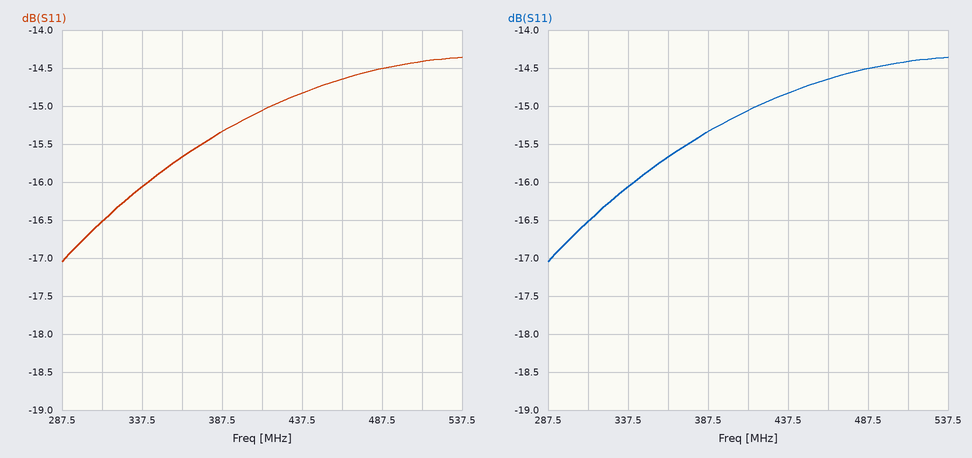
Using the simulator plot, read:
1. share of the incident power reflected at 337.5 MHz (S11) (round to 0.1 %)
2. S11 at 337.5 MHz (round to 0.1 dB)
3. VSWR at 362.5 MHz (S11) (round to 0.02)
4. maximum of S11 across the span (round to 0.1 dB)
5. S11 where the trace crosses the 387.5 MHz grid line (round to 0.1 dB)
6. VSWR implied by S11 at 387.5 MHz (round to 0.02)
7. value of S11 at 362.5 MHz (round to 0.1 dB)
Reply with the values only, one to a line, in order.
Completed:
2.5 %
-16.1 dB
1.40
-14.4 dB
-15.3 dB
1.42
-15.7 dB
